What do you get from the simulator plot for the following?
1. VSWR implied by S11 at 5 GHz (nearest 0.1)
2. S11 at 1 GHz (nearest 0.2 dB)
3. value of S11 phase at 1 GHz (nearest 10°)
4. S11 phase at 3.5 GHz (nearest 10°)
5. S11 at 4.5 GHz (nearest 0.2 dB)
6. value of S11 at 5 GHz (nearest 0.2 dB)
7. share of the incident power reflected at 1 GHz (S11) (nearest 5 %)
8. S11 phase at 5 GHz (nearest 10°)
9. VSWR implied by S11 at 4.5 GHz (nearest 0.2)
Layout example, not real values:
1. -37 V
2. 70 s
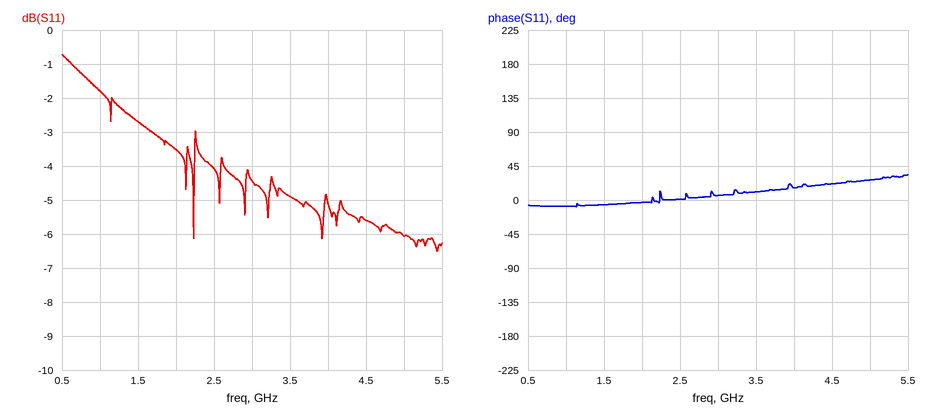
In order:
1. 3.0
2. -1.8 dB
3. -10°
4. 10°
5. -5.6 dB
6. -6.0 dB
7. 65 %
8. 30°
9. 3.2
